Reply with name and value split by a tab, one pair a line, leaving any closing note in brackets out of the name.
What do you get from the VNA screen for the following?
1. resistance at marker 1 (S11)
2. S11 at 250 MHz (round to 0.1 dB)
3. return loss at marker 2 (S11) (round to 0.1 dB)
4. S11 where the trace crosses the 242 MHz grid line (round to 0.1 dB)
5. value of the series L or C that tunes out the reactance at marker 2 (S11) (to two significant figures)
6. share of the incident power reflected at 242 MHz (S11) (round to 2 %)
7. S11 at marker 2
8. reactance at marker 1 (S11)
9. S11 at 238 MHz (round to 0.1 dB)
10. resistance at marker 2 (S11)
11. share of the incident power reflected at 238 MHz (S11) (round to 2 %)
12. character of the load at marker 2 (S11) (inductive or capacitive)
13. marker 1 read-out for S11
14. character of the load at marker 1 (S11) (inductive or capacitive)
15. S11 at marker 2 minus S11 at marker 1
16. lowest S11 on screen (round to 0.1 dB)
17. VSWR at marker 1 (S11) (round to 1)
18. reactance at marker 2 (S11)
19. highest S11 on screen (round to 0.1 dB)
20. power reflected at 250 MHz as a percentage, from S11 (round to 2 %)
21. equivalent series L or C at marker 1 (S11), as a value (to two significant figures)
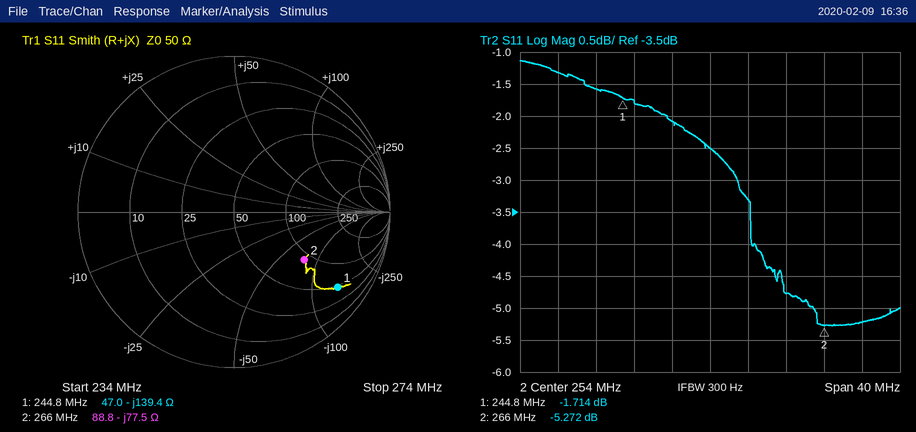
resistance at marker 1	47.0 Ω
S11 at 250 MHz	-2.1 dB
return loss at marker 2 (S11)	5.3 dB
S11 where the trace crosses the 242 MHz grid line	-1.6 dB
value of the series L or C that tunes out the reactance at marker 2 (S11)	46 nH
share of the incident power reflected at 242 MHz (S11)	70 %
S11 at marker 2	-5.272 dB
reactance at marker 1	-139.4 Ω
S11 at 238 MHz	-1.3 dB
resistance at marker 2	88.8 Ω
share of the incident power reflected at 238 MHz (S11)	74 %
character of the load at marker 2 (S11)	capacitive
marker 1 read-out for S11	-1.714 dB
character of the load at marker 1 (S11)	capacitive
S11 at marker 2 minus S11 at marker 1	-3.558 dB
lowest S11 on screen	-5.3 dB
VSWR at marker 1 (S11)	10
reactance at marker 2	-77.5 Ω
highest S11 on screen	-1.1 dB
power reflected at 250 MHz as a percentage, from S11	62 %
equivalent series L or C at marker 1 (S11), as a value	4.7 pF
